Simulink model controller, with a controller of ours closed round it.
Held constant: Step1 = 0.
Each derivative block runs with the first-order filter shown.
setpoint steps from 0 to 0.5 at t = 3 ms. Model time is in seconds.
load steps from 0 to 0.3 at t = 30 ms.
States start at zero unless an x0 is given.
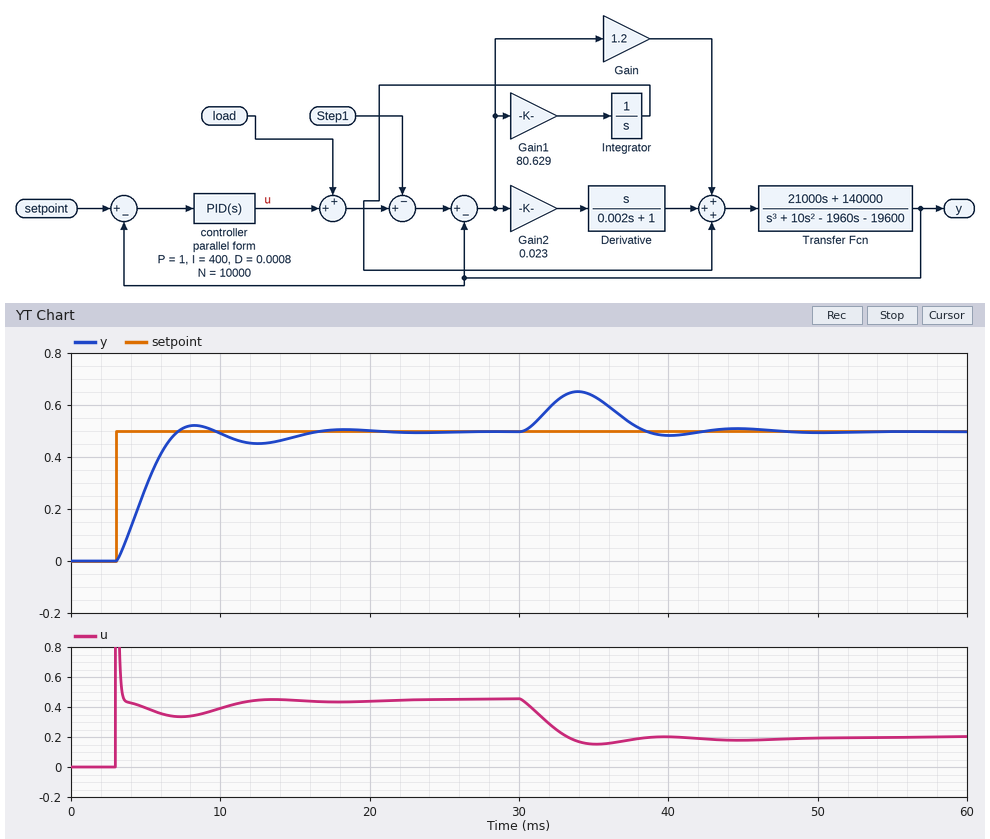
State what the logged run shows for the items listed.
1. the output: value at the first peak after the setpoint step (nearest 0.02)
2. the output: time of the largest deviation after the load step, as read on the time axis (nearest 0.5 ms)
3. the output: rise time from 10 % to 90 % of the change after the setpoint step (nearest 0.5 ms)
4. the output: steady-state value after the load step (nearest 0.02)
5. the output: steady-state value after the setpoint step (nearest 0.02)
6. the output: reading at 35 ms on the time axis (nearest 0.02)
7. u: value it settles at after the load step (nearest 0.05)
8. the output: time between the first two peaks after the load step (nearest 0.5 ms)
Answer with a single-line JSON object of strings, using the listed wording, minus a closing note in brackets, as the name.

{"the output: value at the first peak after the setpoint step": "0.52", "the output: time of the largest deviation after the load step, as read on the time axis": "34.0 ms", "the output: rise time from 10 % to 90 % of the change after the setpoint step": "3.0 ms", "the output: steady-state value after the load step": "0.50", "the output: steady-state value after the setpoint step": "0.50", "the output: reading at 35 ms on the time axis": "0.64", "u: value it settles at after the load step": "0.20", "the output: time between the first two peaks after the load step": "10.5 ms"}
